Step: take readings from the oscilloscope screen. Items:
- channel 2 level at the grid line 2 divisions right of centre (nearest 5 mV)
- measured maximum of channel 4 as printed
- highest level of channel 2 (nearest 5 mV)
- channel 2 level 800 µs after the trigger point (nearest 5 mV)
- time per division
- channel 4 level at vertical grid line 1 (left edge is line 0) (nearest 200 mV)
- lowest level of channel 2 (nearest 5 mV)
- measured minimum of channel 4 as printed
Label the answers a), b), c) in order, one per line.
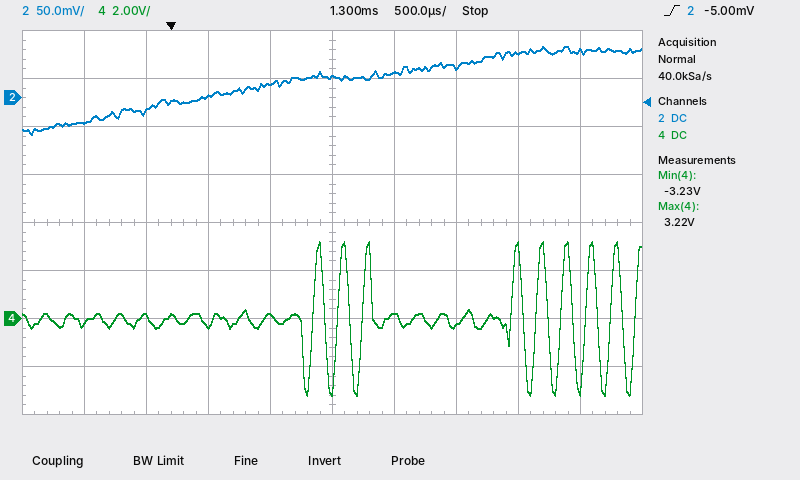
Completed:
a) 30 mV
b) 3.22 V
c) 55 mV
d) 15 mV
e) 500 µs
f) -200 mV
g) -40 mV
h) -3.23 V
